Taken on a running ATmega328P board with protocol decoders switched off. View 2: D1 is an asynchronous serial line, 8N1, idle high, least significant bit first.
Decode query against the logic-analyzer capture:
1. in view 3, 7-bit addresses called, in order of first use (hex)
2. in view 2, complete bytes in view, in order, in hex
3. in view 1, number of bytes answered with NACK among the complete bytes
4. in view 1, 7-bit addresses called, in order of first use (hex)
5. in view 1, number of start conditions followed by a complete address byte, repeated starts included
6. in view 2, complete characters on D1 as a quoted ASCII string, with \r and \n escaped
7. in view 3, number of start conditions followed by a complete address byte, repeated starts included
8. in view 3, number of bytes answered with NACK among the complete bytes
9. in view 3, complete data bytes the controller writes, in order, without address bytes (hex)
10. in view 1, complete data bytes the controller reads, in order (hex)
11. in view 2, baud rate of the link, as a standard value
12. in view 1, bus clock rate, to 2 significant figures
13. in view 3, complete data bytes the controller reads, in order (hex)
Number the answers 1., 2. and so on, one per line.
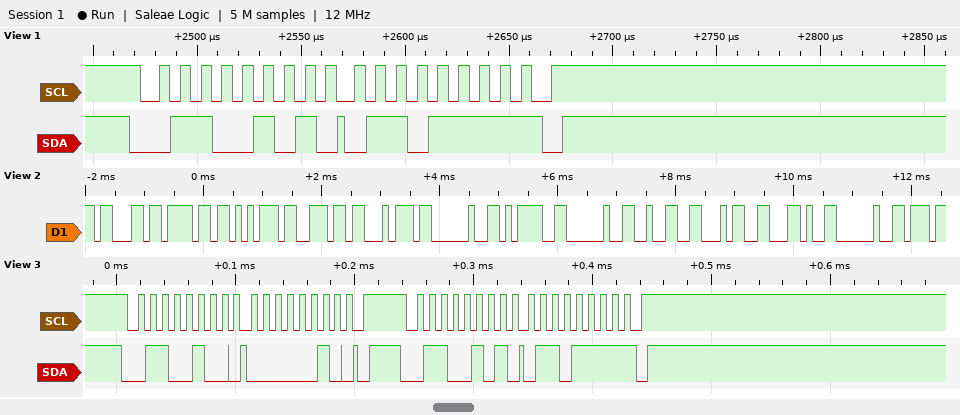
1. 0x32
2. 63 6F 75 6E 74 20 3D 20 32 34 2C 20
3. 1
4. 0x32
5. 1
6. "count = 24, "
7. 2
8. 1
9. 02
10. 6F
11. 9600 baud
12. 100 kHz
13. 6F
